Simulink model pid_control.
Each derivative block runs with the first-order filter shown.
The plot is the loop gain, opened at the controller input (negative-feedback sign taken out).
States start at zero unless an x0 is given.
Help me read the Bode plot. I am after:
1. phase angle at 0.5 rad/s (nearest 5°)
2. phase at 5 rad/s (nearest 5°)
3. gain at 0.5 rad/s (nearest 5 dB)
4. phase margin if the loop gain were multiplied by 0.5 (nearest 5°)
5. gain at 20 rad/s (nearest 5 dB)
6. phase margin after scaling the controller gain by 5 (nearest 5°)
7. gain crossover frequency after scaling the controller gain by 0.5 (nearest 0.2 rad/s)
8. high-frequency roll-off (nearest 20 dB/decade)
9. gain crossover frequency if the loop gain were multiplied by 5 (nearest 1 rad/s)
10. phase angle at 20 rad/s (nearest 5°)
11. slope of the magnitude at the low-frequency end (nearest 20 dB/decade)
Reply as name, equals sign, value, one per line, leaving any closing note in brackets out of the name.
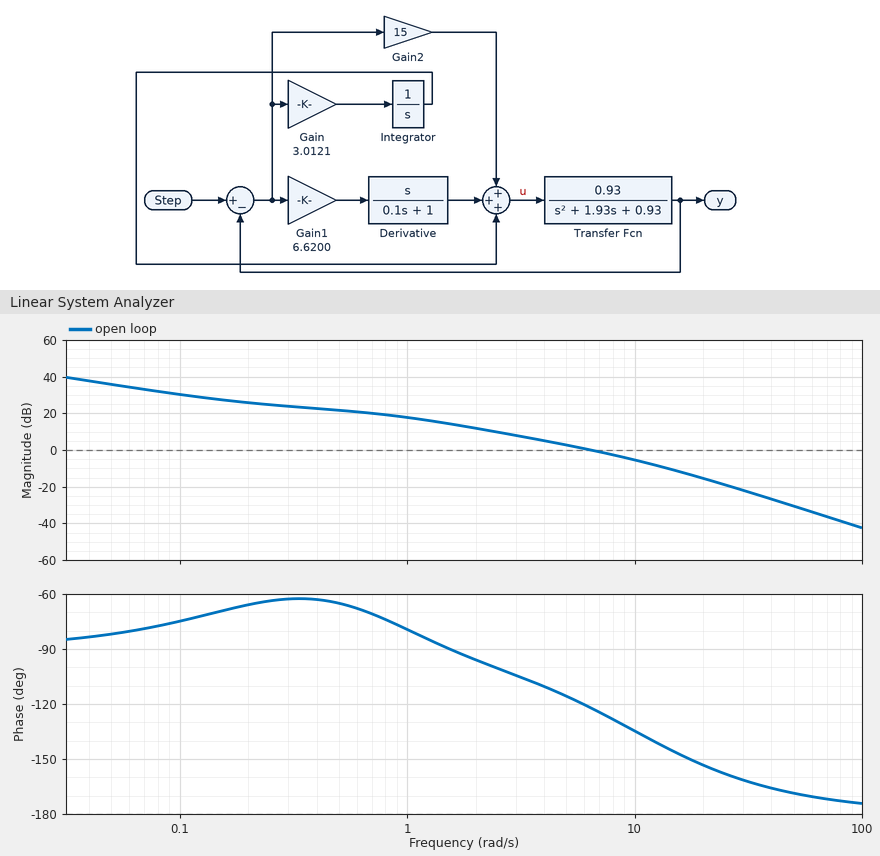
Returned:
phase angle at 0.5 rad/s = -65°
phase at 5 rad/s = -115°
gain at 0.5 rad/s = 20 dB
phase margin if the loop gain were multiplied by 0.5 = 70°
gain at 20 rad/s = -15 dB
phase margin after scaling the controller gain by 5 = 30°
gain crossover frequency after scaling the controller gain by 0.5 = 3.6 rad/s
high-frequency roll-off = -40 dB/decade
gain crossover frequency if the loop gain were multiplied by 5 = 18 rad/s
phase angle at 20 rad/s = -155°
slope of the magnitude at the low-frequency end = -20 dB/decade
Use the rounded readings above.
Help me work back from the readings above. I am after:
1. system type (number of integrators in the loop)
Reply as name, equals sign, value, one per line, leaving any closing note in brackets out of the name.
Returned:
system type = 1
